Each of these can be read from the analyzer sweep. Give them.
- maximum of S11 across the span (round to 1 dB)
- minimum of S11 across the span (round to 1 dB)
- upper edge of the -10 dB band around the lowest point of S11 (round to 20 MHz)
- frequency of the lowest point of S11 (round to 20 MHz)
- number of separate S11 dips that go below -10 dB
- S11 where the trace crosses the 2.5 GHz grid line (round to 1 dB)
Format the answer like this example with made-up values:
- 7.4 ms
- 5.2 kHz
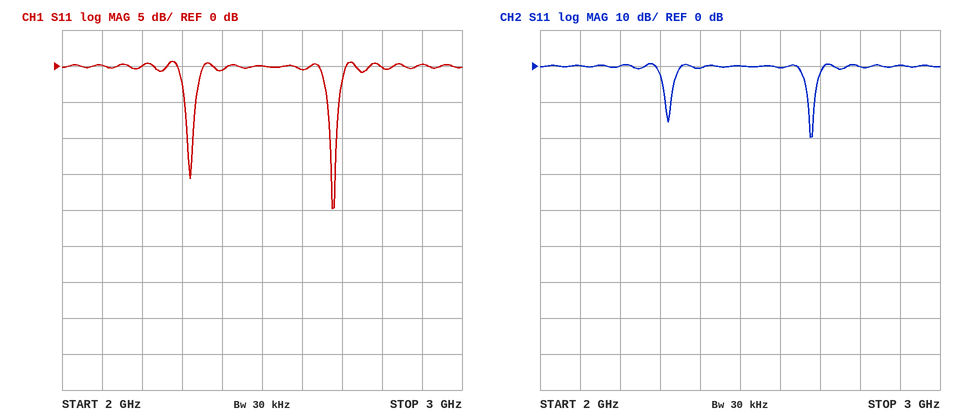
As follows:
- 1 dB
- -20 dB
- 2.68 GHz
- 2.68 GHz
- 2
- 0 dB
